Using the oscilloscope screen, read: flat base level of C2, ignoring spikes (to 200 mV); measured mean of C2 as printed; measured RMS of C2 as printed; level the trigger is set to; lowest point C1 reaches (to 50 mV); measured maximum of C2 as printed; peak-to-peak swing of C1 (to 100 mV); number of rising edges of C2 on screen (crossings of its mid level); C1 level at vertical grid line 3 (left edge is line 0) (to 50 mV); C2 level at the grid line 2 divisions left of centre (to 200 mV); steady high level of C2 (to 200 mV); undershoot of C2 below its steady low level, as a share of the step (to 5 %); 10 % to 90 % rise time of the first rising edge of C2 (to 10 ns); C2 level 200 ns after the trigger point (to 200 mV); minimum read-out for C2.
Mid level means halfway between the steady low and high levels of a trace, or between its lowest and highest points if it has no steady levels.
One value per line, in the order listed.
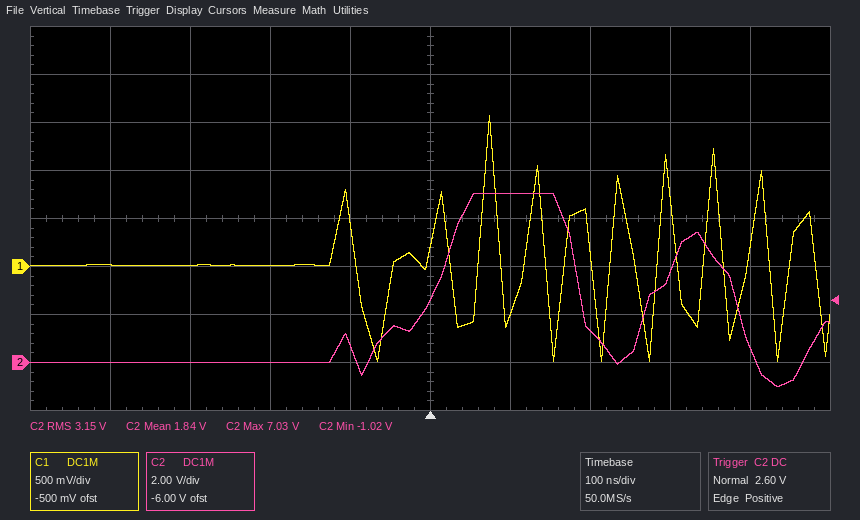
0.0 V
1.84 V
3.15 V
2.60 V
-1.00 V
7.03 V
2.60 V
2
0 mV
0.0 V
7.0 V
15 %
110 ns
1.4 V
-1.02 V
